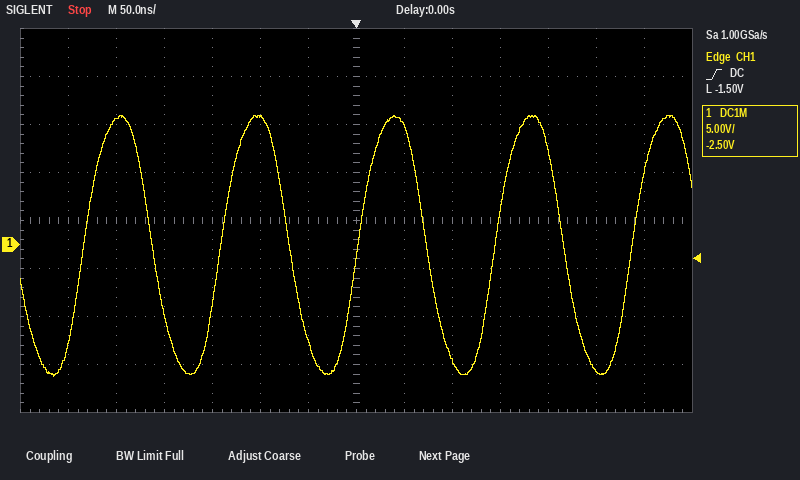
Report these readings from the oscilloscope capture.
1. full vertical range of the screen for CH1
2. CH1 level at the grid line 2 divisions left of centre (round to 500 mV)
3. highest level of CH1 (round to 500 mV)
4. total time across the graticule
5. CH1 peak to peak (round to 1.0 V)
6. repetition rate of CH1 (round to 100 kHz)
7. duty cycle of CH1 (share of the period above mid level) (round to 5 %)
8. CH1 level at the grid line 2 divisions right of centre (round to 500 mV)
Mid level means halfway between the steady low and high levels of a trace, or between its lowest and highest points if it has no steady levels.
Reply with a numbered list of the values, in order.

1. 40 V
2. 13.5 V
3. 13.5 V
4. 700 ns
5. 27.0 V
6. 7.0 MHz
7. 50 %
8. -12.0 V
